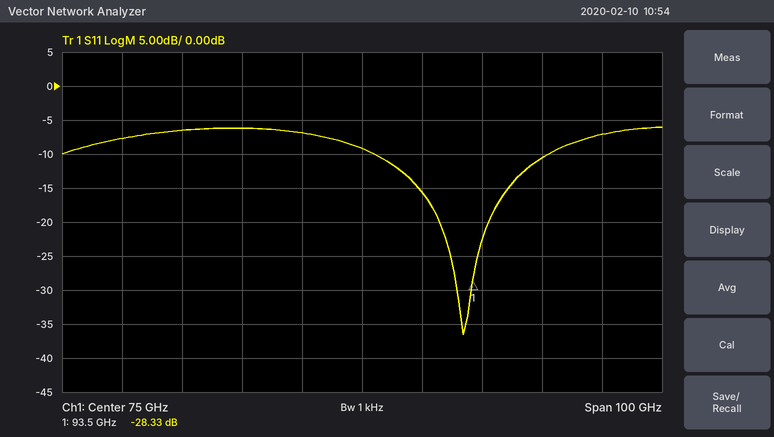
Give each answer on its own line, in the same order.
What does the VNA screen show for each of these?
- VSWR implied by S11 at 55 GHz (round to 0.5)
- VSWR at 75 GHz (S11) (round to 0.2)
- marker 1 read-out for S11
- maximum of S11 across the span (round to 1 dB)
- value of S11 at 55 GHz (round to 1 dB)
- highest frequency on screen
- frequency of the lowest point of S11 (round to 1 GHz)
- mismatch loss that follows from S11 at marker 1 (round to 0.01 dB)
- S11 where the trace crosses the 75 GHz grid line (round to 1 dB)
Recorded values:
3.0
2.0
-28.33 dB
-6 dB
-6 dB
125 GHz
92 GHz
0.01 dB
-9 dB
